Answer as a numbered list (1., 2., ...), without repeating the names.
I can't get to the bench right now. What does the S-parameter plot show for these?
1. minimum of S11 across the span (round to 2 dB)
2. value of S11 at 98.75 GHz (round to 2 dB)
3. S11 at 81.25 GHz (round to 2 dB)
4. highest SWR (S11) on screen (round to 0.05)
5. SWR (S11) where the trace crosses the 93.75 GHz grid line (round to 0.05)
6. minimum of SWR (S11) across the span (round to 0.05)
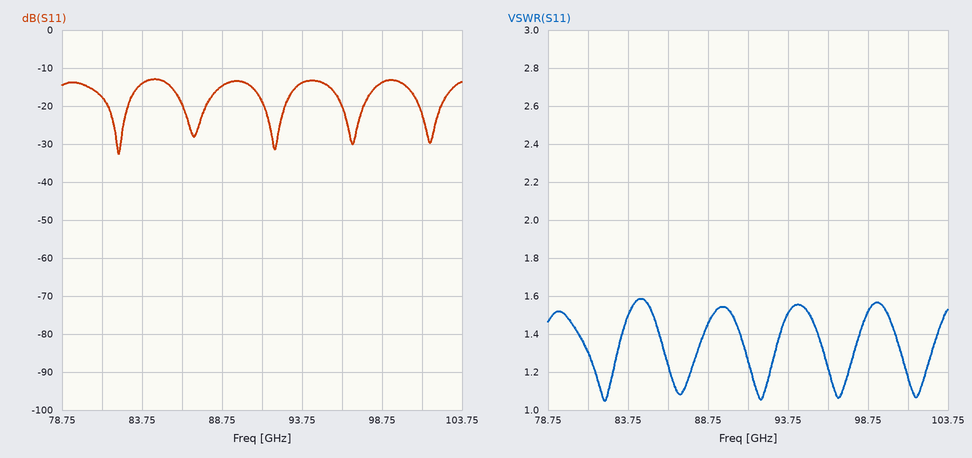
1. -32 dB
2. -14 dB
3. -18 dB
4. 1.60
5. 1.50
6. 1.05
